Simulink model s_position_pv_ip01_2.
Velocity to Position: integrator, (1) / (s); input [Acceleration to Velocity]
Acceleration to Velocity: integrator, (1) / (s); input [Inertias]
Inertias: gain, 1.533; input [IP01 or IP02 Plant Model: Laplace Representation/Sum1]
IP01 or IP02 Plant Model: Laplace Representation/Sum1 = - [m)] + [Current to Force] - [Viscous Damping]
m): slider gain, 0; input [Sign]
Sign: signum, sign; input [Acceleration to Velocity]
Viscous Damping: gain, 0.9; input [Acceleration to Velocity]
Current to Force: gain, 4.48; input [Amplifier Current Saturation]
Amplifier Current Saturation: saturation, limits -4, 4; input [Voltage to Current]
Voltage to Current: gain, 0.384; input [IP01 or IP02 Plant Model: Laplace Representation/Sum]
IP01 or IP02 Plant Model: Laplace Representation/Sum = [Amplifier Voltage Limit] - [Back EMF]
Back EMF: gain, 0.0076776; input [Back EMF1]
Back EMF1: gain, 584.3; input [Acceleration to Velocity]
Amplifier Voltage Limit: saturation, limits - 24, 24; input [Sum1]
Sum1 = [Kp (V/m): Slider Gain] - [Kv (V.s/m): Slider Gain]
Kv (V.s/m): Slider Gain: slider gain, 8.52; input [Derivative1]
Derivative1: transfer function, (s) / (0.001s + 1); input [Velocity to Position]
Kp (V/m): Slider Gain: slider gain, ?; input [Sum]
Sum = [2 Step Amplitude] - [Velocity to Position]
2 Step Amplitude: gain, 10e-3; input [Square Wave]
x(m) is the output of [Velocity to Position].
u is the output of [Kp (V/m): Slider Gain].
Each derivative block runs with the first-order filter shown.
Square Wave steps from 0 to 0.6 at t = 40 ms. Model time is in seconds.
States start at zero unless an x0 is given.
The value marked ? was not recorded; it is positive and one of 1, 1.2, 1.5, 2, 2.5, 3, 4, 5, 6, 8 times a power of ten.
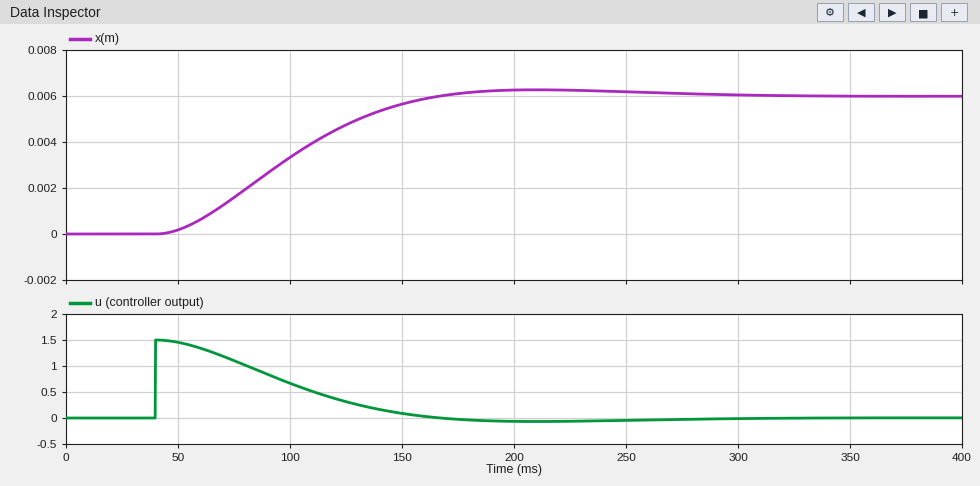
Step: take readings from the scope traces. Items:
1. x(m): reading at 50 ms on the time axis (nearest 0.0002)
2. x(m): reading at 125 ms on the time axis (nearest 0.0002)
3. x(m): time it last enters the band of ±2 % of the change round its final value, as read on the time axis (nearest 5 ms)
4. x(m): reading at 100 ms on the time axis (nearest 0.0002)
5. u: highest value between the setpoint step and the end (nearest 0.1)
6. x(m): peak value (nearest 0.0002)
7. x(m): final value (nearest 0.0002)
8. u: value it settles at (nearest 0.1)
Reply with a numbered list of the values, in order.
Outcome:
1. 0.0002
2. 0.0048
3. 270 ms
4. 0.0034
5. 1.5
6. 0.0062
7. 0.0060
8. 0.0
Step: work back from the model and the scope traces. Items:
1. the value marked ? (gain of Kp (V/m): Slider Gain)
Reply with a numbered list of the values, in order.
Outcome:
1. 250
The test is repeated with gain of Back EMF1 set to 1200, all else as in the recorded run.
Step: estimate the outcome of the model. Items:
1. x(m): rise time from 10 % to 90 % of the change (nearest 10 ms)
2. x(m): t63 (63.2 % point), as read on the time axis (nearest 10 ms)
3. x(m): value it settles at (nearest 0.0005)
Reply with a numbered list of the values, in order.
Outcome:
1. 120 ms
2. 120 ms
3. 0.0060
